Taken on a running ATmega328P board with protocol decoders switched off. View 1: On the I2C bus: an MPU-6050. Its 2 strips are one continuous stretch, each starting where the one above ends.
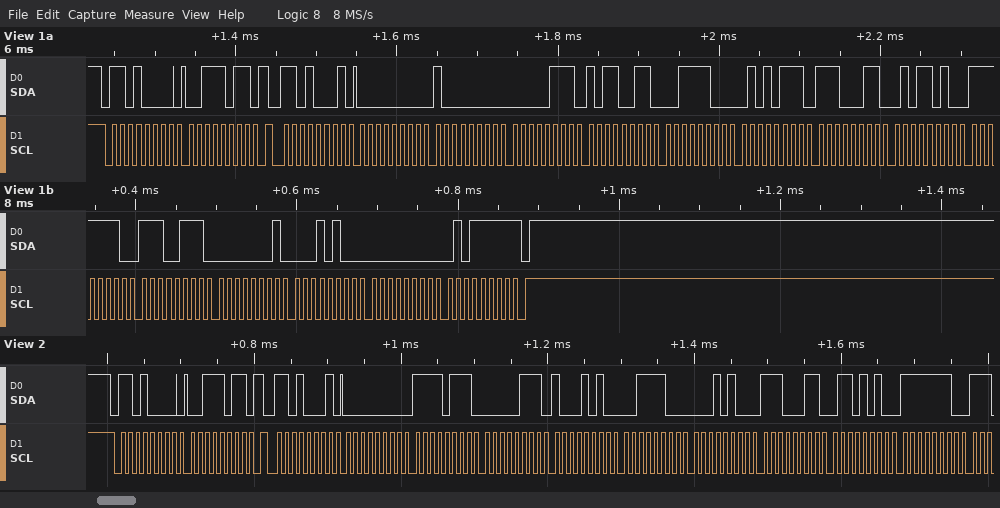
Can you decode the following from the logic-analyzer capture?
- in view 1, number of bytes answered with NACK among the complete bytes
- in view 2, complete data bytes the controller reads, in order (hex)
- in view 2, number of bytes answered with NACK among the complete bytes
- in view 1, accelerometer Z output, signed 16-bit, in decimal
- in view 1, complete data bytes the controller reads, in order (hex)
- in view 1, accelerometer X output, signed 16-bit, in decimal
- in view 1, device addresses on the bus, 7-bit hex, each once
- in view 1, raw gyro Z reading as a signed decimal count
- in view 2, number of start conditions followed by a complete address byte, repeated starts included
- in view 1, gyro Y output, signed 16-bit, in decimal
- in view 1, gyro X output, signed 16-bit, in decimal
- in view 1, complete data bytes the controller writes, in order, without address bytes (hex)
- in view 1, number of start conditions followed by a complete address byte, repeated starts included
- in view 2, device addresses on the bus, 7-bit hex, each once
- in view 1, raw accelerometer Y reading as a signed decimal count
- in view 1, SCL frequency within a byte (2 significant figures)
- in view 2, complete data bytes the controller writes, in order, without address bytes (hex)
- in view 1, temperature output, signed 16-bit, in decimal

1
00 F7 07 8A 3C 14 E3 6A FE
0
15447
00 80 07 B3 3C 57 E3 5A FE E7 01 14 00 5F
128
0x68
95
2
276
-281
3B
2
0x68
1971
100 kHz
3B
-7334
